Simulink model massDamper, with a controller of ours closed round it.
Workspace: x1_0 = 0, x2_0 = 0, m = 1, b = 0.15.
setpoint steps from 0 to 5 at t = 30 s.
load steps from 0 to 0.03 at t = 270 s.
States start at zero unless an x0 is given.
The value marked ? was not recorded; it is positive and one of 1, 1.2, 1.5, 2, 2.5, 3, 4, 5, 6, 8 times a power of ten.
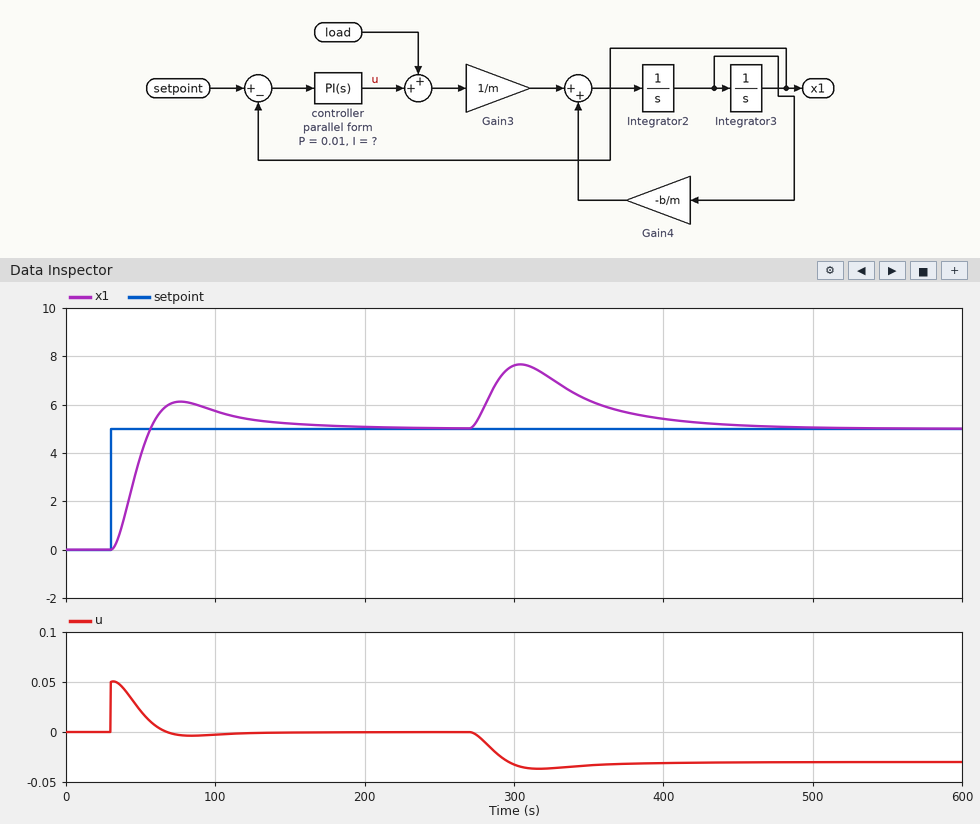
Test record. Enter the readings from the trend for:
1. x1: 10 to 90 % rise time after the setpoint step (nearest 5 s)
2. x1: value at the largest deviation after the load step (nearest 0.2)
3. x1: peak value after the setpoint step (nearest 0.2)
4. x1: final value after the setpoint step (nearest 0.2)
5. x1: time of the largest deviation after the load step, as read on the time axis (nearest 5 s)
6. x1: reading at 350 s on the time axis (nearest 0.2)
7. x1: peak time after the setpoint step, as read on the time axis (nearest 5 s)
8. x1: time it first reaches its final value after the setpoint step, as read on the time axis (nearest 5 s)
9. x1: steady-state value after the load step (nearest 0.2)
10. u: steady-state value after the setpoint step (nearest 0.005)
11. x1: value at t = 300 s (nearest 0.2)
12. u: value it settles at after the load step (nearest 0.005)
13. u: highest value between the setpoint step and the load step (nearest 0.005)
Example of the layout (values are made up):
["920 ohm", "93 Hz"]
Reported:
["20 s", "7.6", "6.2", "5.0", "305 s", "6.2", "75 s", "55 s", "5.0", "0.000", "7.6", "-0.030", "0.050"]
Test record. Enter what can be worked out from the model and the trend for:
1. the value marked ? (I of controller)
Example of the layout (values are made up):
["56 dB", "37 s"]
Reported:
["0.00015"]
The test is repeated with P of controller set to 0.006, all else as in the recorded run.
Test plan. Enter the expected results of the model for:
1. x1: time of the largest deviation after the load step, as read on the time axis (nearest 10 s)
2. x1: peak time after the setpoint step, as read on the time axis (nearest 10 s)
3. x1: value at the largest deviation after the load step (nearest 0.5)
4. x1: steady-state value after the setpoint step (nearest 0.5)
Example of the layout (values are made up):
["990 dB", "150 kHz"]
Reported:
["310 s", "100 s", "8.5", "5.0"]
